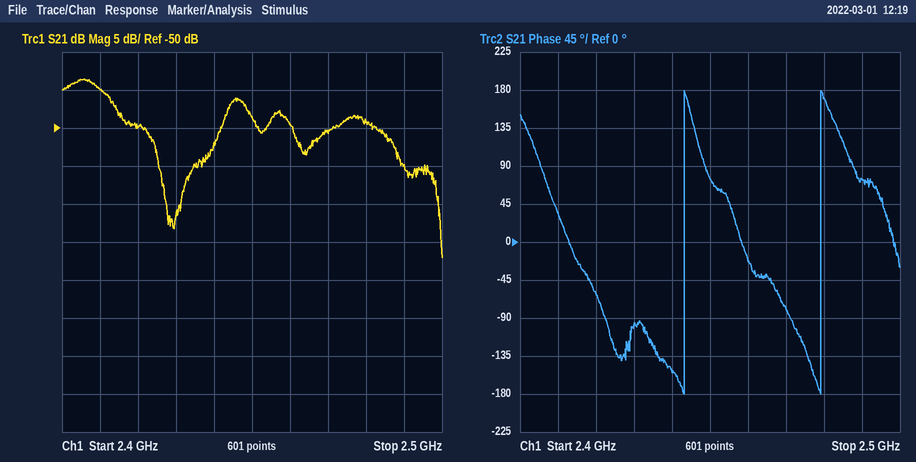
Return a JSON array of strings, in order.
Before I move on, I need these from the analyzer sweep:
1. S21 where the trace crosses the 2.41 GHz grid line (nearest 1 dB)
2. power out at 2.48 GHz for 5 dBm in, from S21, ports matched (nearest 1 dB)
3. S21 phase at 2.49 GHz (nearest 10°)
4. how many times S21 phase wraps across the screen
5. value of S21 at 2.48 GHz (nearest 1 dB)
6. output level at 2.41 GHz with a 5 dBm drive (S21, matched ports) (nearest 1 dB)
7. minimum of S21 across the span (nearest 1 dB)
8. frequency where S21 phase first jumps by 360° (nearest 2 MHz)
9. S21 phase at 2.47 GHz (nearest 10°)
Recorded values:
["-45 dB", "-44 dBm", "70°", "2", "-49 dB", "-40 dBm", "-67 dB", "2.444 GHz", "-80°"]
